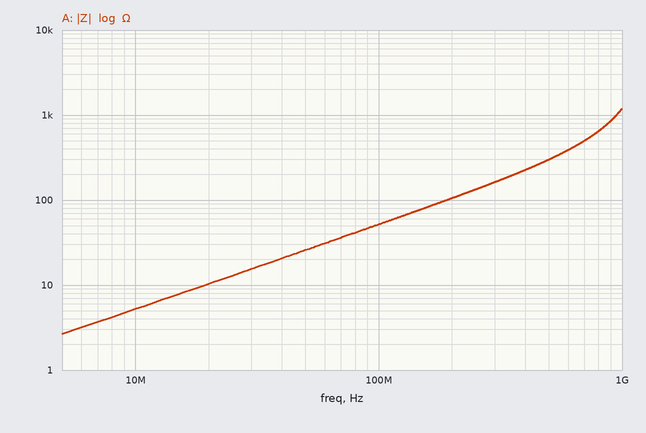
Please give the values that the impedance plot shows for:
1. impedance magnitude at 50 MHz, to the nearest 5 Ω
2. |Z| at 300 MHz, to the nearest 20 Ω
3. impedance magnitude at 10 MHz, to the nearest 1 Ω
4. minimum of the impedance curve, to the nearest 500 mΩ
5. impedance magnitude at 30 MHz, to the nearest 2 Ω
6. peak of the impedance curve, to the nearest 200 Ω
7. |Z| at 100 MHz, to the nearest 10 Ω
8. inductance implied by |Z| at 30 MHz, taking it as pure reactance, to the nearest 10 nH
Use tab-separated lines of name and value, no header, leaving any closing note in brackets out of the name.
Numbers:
impedance magnitude at 50 MHz, to the nearest 5 Ω	25 Ω
|Z| at 300 MHz, to the nearest 20 Ω	160 Ω
impedance magnitude at 10 MHz, to the nearest 1 Ω	5 Ω
minimum of the impedance curve, to the nearest 500 mΩ	2.5 Ω
impedance magnitude at 30 MHz, to the nearest 2 Ω	16 Ω
peak of the impedance curve, to the nearest 200 Ω	1.2 kΩ
|Z| at 100 MHz, to the nearest 10 Ω	50 Ω
inductance implied by |Z| at 30 MHz, taking it as pure reactance, to the nearest 10 nH	80 nH
